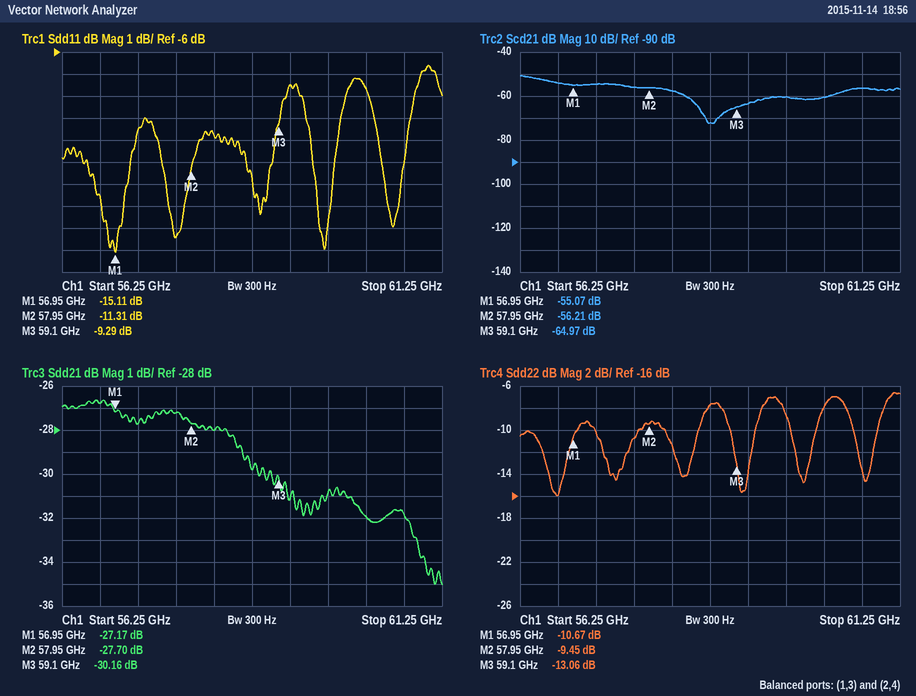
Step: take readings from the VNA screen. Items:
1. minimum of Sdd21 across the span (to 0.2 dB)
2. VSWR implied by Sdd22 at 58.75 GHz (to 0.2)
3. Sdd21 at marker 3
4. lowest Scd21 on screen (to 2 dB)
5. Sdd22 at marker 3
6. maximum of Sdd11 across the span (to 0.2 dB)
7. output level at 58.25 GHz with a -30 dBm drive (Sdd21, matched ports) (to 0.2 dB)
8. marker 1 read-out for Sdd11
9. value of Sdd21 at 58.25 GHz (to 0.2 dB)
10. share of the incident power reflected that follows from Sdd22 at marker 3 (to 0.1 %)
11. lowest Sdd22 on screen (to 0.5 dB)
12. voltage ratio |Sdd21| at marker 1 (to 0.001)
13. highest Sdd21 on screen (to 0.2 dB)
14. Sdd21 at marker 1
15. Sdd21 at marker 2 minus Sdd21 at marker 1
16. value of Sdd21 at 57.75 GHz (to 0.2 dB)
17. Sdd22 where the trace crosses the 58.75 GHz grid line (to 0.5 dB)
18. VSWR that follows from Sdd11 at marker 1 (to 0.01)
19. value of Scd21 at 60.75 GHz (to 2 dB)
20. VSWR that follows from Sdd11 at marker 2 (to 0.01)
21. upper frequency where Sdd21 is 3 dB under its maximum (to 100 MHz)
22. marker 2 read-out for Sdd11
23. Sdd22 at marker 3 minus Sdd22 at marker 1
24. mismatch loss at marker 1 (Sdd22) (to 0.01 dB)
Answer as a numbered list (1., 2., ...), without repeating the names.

1. -35.0 dB
2. 2.4
3. -30.16 dB
4. -72 dB
5. -13.06 dB
6. -6.6 dB
7. -58.0 dBm
8. -15.11 dB
9. -28.0 dB
10. 4.9 %
11. -16.0 dB
12. 0.044
13. -26.6 dB
14. -27.17 dB
15. -0.53 dB
16. -27.2 dB
17. -7.5 dB
18. 1.43
19. -56 dB
20. 1.75
21. 58.7 GHz
22. -11.31 dB
23. -2.39 dB
24. 0.39 dB
